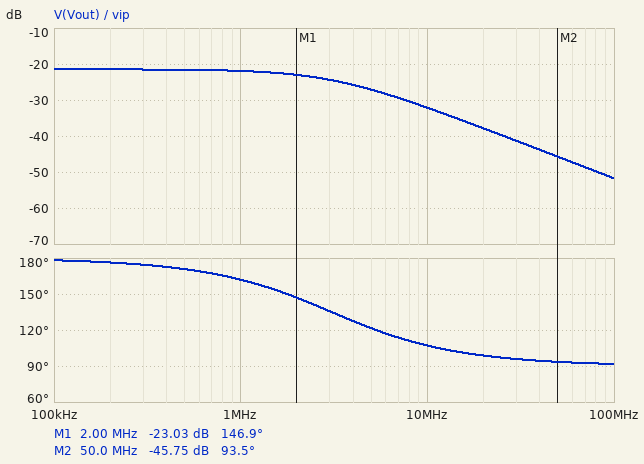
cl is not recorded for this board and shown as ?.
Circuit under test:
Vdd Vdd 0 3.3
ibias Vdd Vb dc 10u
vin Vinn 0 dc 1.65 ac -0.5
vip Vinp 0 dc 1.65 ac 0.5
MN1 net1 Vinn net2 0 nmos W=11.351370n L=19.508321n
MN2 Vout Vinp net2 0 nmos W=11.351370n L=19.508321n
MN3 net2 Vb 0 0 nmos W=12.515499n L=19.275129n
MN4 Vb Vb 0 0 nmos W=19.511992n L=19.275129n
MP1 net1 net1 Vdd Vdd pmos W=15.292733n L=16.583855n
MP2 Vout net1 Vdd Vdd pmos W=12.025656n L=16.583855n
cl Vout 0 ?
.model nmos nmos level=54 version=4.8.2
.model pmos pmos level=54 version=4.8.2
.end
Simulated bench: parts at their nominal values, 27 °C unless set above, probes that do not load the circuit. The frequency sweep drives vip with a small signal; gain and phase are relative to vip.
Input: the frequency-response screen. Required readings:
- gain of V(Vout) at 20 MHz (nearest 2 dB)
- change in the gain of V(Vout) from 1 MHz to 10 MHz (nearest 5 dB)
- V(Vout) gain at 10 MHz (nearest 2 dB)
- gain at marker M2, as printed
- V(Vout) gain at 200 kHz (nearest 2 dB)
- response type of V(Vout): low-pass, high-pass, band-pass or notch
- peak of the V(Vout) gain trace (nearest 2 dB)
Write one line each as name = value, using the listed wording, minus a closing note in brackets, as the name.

gain of V(Vout) at 20 MHz = -38 dB
change in the gain of V(Vout) from 1 MHz to 10 MHz = -10 dB
V(Vout) gain at 10 MHz = -32 dB
gain at marker M2, as printed = -45.75 dB
V(Vout) gain at 200 kHz = -22 dB
response type of V(Vout): low-pass, high-pass, band-pass or notch = low-pass
peak of the V(Vout) gain trace = -22 dB
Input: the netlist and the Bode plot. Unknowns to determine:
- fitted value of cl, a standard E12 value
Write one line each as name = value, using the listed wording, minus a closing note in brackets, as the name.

fitted value of cl, a standard E12 value = 6.8 pF
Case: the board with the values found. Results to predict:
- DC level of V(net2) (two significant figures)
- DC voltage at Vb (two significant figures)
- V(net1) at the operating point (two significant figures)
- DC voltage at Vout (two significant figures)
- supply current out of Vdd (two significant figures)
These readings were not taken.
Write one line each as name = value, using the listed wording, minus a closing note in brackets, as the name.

DC level of V(net2) = 2.2 V
DC voltage at Vb = 50 mV
V(net1) at the operating point = 2.7 V
DC voltage at Vout = 2.7 V
supply current out of Vdd = 150 µA
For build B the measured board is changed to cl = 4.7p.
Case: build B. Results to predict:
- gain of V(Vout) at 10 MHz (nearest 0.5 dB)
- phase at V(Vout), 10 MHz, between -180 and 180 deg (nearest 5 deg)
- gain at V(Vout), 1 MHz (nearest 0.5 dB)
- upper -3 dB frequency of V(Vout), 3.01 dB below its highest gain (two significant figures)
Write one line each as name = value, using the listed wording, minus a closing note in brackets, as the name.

gain of V(Vout) at 10 MHz = -29.5 dB
phase at V(Vout), 10 MHz, between -180 and 180 deg = 115 deg
gain at V(Vout), 1 MHz = -21.5 dB
upper -3 dB frequency of V(Vout), 3.01 dB below its highest gain = 4.4 MHz
